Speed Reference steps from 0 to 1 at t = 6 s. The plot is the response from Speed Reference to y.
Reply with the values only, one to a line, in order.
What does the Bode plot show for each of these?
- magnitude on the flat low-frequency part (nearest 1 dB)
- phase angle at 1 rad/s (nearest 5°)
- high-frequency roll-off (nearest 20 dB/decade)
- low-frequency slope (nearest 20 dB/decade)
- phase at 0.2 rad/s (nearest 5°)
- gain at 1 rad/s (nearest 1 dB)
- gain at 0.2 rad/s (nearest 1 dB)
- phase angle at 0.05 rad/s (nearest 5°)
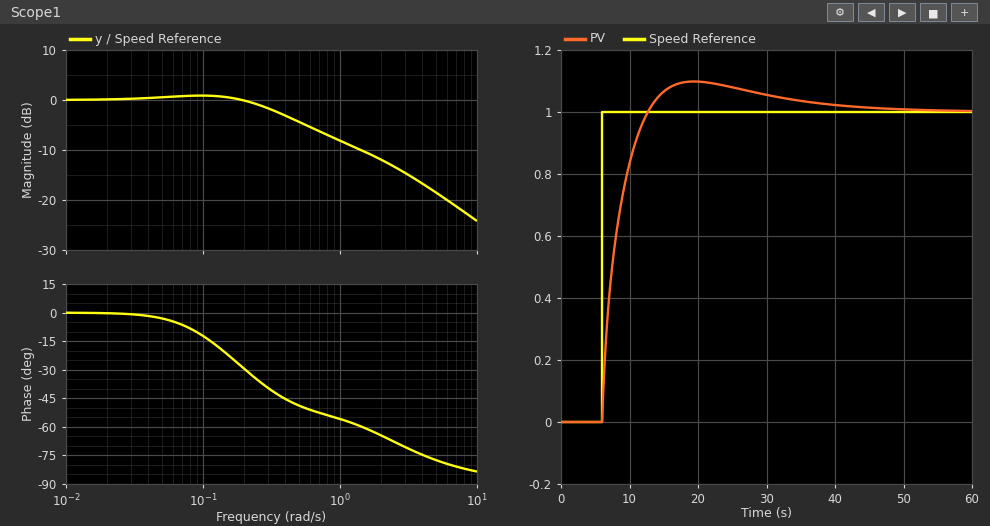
0 dB
-55°
-20 dB/decade
0 dB/decade
-30°
-8 dB
0 dB
-5°
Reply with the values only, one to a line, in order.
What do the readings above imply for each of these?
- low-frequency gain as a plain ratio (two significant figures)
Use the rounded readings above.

1.0
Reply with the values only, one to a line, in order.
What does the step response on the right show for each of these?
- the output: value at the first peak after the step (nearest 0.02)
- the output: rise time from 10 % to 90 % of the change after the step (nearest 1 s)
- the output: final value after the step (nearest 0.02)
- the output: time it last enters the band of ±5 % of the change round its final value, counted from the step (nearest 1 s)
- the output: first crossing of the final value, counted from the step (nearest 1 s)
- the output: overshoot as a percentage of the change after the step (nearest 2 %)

1.10
5 s
1.00
25 s
7 s
10 %
